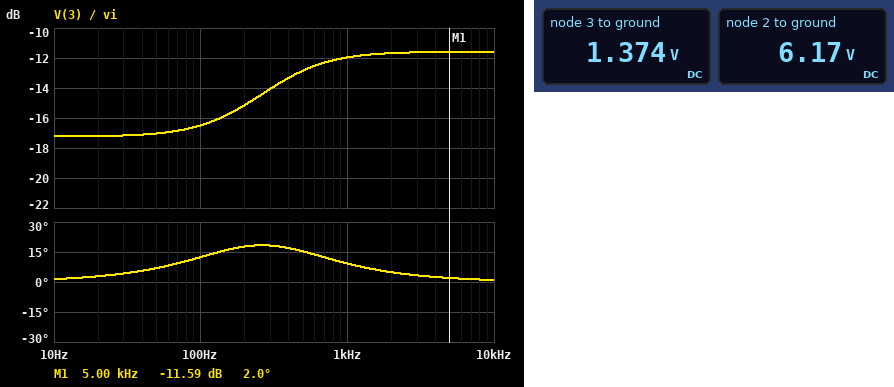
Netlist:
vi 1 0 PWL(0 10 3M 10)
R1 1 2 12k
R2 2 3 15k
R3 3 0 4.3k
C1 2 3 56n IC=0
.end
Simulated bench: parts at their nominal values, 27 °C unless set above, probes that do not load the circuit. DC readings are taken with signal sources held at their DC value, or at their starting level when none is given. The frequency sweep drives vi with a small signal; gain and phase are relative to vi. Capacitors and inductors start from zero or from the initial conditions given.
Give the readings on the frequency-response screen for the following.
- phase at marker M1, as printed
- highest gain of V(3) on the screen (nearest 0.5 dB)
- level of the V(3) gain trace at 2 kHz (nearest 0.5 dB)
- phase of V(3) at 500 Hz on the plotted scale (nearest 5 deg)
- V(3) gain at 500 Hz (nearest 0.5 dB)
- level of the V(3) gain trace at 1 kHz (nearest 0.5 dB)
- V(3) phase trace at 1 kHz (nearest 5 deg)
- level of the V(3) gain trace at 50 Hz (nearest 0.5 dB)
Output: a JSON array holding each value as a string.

["2.0 deg", "-11.5 dB", "-11.5 dB", "15 deg", "-13.0 dB", "-12.0 dB", "10 deg", "-17.0 dB"]
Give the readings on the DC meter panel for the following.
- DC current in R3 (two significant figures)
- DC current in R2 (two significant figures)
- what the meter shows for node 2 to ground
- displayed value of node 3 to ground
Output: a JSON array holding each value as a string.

["320 µA", "320 µA", "6.17 V", "1.374 V"]
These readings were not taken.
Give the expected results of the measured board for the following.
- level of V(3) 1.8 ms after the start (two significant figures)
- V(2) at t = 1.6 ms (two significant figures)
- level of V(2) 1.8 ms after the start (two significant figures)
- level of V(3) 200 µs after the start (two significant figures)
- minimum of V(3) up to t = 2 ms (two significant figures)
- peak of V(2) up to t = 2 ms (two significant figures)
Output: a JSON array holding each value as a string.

["1.4 V", "6.1 V", "6.1 V", "2.2 V", "1.4 V", "6.1 V"]
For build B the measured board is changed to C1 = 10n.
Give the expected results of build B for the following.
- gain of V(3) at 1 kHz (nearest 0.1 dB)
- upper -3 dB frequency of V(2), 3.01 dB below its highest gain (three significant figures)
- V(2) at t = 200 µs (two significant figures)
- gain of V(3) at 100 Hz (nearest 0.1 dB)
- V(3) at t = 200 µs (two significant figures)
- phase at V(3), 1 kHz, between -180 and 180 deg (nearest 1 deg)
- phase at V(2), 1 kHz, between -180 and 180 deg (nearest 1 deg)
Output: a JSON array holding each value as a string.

["-15.4 dB", "2.56 kHz", "5.9 V", "-17.2 dB", "1.5 V", "17 deg", "-14 deg"]
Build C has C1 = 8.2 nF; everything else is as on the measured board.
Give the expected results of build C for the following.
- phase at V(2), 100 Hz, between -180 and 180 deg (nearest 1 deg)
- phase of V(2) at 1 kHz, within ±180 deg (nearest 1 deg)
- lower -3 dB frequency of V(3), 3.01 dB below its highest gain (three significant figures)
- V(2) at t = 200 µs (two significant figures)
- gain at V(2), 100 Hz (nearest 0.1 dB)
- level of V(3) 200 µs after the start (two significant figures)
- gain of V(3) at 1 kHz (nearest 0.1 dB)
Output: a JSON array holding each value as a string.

["-1 deg", "-12 deg", "1.68 kHz", "6.0 V", "-4.2 dB", "1.4 V", "-15.9 dB"]
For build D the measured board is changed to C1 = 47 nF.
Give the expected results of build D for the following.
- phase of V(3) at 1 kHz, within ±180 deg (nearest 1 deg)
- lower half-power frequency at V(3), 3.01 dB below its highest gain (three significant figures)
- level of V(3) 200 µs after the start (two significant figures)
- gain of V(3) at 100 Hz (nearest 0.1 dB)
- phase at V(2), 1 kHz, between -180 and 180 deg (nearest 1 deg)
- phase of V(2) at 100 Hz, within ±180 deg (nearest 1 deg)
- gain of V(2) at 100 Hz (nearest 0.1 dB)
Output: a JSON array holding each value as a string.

["11 deg", "293 Hz", "2.1 V", "-16.7 dB", "-22 deg", "-7 deg", "-4.4 dB"]
